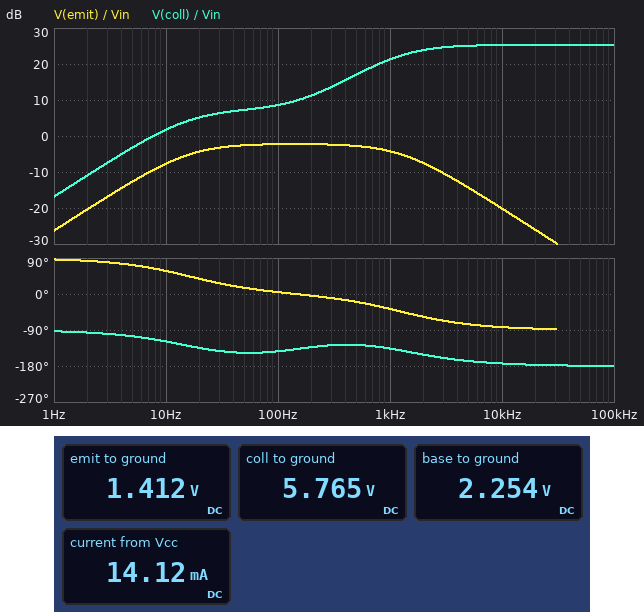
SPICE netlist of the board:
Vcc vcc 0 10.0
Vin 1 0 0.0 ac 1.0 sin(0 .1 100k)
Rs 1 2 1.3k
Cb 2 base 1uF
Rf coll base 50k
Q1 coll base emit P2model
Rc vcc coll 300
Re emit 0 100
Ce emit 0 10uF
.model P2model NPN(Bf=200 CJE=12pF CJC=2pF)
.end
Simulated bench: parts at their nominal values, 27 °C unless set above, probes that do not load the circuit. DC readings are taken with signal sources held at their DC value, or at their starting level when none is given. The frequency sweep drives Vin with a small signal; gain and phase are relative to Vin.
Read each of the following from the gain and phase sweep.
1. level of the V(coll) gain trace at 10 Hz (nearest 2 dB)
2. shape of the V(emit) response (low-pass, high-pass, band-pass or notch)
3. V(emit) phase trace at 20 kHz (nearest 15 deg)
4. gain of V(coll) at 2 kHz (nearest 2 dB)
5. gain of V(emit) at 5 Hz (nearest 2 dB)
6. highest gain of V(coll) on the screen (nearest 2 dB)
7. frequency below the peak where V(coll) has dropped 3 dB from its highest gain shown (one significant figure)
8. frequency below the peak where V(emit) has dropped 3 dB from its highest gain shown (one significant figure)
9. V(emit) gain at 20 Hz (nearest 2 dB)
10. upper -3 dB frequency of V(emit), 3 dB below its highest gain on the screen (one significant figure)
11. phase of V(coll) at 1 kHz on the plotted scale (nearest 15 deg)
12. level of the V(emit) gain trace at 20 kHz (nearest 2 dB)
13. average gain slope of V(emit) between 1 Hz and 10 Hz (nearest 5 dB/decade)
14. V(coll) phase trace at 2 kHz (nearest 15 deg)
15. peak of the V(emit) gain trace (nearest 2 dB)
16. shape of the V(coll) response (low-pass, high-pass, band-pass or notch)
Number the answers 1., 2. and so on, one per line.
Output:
1. 2 dB
2. band-pass
3. -90 deg
4. 24 dB
5. -12 dB
6. 26 dB
7. 1 kHz
8. 20 Hz
9. -4 dB
10. 1 kHz
11. -135 deg
12. -26 dB
13. 20 dB/decade
14. -150 deg
15. -2 dB
16. high-pass
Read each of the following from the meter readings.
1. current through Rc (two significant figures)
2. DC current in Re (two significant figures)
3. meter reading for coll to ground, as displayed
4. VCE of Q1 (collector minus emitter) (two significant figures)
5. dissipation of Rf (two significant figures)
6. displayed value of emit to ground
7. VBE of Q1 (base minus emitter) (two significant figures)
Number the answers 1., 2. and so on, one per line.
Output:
1. 14 mA
2. 14 mA
3. 5.765 V
4. 4.4 V
5. 250 µW
6. 1.412 V
7. 840 mV
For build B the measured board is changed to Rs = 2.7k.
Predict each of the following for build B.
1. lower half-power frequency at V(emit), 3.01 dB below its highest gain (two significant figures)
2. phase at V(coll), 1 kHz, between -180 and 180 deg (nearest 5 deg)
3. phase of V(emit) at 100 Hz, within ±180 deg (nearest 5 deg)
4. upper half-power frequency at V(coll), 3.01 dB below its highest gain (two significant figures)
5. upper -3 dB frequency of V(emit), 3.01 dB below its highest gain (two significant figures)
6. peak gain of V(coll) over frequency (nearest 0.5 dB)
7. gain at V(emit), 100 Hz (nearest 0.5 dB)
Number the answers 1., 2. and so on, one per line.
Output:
1. 14 Hz
2. -150 deg
3. 0 deg
4. 4.9 MHz
5. 760 Hz
6. 19.5 dB
7. -3.5 dB
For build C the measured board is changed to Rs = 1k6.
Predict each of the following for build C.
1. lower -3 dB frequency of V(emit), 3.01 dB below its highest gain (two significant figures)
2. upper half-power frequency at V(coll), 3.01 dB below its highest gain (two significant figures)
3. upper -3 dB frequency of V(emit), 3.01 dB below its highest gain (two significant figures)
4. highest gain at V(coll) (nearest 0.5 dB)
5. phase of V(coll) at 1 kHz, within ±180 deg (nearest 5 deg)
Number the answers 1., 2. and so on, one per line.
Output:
1. 15 Hz
2. 5.1 MHz
3. 1.1 kHz
4. 23.5 dB
5. -140 deg
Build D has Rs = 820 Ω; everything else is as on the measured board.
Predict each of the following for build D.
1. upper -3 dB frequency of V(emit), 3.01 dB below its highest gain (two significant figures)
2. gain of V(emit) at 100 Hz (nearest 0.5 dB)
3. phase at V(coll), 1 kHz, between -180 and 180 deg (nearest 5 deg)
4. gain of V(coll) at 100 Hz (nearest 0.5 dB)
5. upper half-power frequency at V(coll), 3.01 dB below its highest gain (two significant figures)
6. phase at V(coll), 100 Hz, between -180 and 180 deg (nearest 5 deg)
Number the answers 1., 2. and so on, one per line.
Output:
1. 1.8 kHz
2. -2.0 dB
3. -125 deg
4. 9.0 dB
5. 5.6 MHz
6. -140 deg
